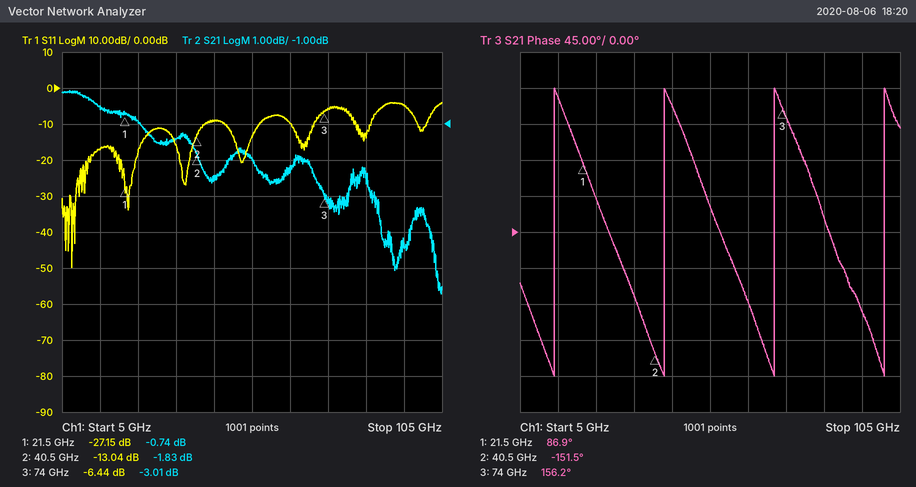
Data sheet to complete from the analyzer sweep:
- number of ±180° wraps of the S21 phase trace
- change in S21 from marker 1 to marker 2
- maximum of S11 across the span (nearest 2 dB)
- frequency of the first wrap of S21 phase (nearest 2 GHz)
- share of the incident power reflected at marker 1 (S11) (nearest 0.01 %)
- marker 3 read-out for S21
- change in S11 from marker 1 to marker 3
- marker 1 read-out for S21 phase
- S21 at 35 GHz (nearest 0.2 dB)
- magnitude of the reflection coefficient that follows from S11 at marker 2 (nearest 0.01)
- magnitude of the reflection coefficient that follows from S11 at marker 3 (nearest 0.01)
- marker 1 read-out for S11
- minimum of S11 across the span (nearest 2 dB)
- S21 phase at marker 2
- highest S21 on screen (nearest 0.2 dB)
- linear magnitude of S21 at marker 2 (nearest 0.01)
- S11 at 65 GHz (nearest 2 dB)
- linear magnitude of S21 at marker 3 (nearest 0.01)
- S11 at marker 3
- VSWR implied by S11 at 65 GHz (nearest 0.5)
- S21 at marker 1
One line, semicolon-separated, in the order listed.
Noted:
4; -1.09 dB; -4 dB; 14 GHz; 0.19 %; -3.01 dB; 20.71 dB; 86.9°; -1.4 dB; 0.22; 0.48; -27.15 dB; -50 dB; -151.5°; 0.0 dB; 0.81; -10 dB; 0.71; -6.44 dB; 2.0; -0.74 dB
